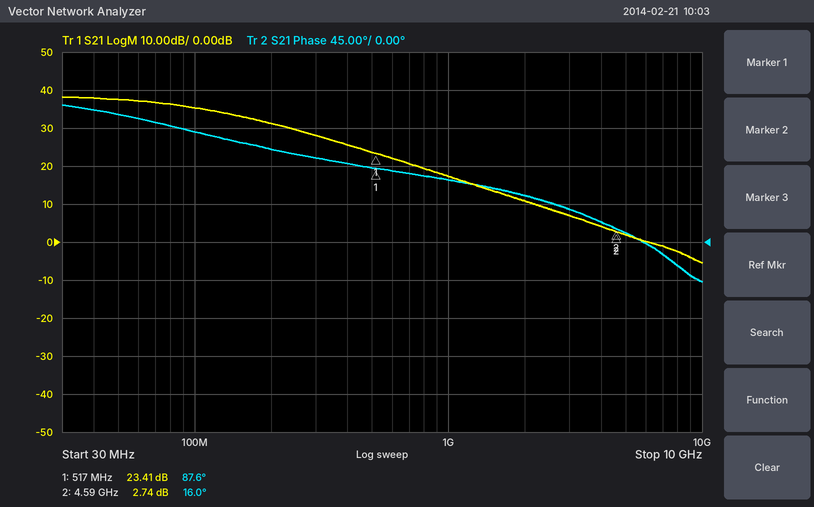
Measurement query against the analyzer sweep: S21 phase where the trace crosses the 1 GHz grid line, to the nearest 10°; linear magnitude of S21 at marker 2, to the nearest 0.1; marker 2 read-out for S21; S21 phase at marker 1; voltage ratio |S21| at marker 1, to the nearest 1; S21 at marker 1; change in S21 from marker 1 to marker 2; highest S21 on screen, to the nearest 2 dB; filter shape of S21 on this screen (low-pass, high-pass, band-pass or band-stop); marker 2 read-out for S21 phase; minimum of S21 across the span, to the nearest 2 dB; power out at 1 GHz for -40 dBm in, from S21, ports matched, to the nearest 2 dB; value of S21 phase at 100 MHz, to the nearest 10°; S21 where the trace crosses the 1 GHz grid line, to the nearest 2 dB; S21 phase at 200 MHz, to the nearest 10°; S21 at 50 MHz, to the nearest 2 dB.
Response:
70°
1.4
2.74 dB
87.6°
15
23.41 dB
-20.67 dB
38 dB
low-pass
16.0°
-6 dB
-22 dBm
130°
18 dB
110°
38 dB
